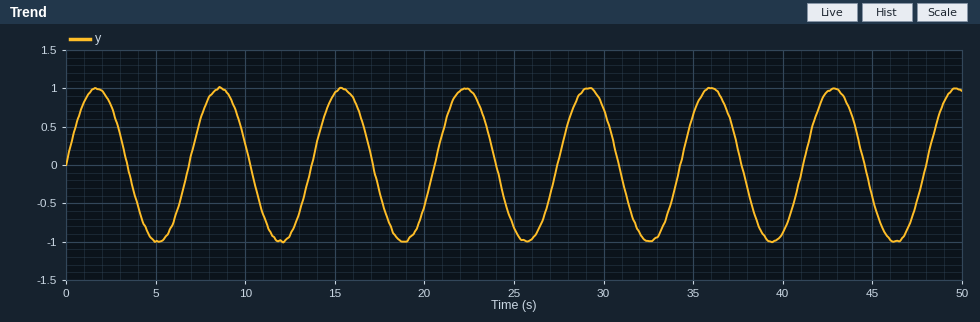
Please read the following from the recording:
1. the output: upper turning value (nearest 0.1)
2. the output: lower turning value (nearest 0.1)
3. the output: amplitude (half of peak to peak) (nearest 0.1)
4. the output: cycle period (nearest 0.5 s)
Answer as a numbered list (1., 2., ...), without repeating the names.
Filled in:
1. 1.0
2. -1.0
3. 1.0
4. 7.0 s
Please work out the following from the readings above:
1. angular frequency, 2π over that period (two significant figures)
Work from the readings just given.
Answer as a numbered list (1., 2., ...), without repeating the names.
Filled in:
1. 0.90 rad/s
